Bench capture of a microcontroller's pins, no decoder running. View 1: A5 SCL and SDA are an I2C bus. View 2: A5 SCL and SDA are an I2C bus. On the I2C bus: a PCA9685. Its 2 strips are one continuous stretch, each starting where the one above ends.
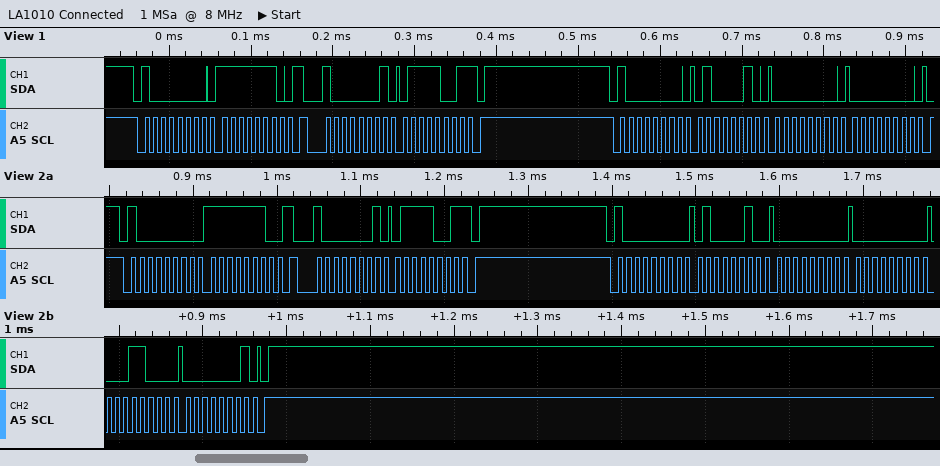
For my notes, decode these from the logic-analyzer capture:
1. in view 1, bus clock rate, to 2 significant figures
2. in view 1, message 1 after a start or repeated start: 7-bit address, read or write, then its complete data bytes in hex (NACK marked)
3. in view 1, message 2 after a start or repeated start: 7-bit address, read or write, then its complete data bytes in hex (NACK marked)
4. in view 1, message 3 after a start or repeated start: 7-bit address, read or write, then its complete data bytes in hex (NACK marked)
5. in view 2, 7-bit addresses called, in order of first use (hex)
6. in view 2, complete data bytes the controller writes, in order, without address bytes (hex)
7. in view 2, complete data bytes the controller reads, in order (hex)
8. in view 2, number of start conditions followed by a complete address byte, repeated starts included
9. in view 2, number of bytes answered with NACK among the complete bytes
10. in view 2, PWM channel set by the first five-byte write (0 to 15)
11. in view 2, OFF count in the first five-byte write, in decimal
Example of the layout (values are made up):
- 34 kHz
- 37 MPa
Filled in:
- 100 kHz
- 0x40 write: FE
- 0x40 read: 79 NACK
- 0x40 write: 42 00 00
- 0x40
- FE 42 00 00 18 01
- 79
- 3
- 1
- 15
- 280
